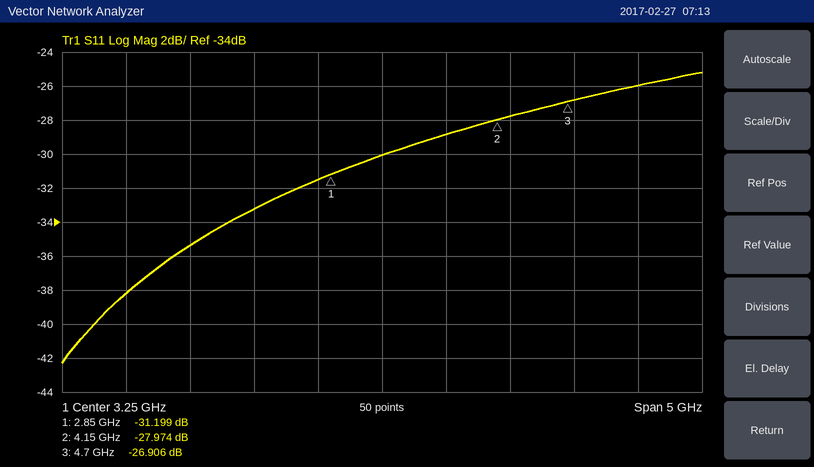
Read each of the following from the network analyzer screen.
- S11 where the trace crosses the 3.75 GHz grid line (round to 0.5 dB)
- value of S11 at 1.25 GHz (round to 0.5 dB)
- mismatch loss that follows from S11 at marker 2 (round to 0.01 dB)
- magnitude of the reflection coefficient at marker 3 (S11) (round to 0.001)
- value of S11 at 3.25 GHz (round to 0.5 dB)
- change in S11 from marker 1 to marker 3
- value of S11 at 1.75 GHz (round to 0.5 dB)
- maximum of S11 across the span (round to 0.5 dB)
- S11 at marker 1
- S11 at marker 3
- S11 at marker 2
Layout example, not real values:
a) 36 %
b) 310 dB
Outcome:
a) -29.0 dB
b) -38.0 dB
c) 0.01 dB
d) 0.045
e) -30.0 dB
f) 4.293 dB
g) -35.5 dB
h) -25.0 dB
i) -31.199 dB
j) -26.906 dB
k) -27.974 dB
